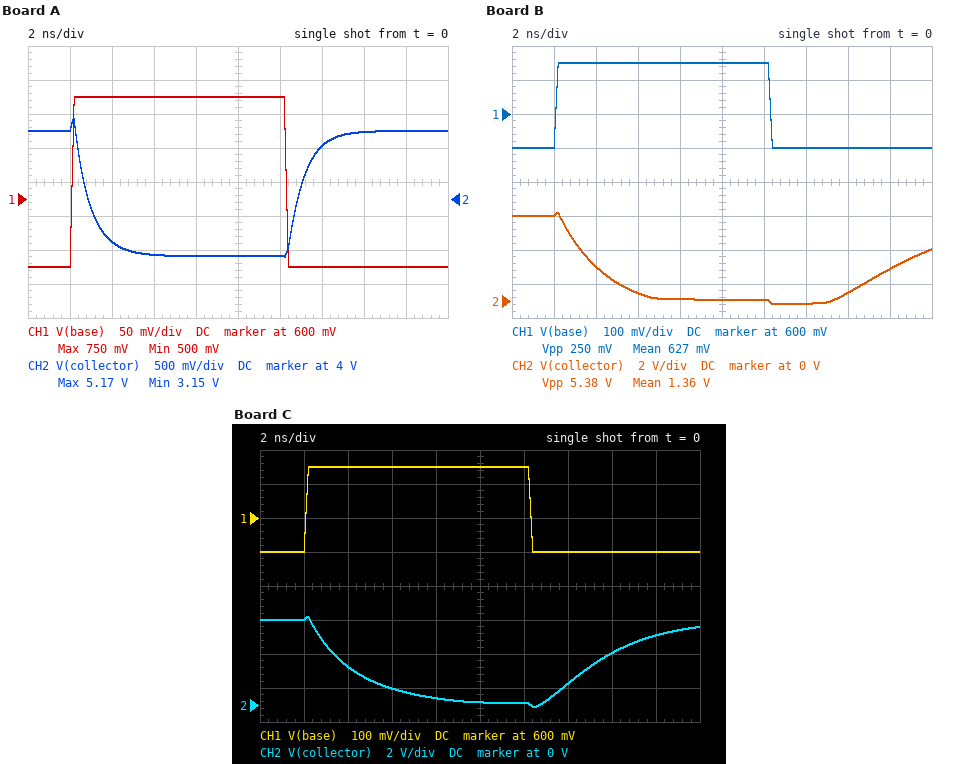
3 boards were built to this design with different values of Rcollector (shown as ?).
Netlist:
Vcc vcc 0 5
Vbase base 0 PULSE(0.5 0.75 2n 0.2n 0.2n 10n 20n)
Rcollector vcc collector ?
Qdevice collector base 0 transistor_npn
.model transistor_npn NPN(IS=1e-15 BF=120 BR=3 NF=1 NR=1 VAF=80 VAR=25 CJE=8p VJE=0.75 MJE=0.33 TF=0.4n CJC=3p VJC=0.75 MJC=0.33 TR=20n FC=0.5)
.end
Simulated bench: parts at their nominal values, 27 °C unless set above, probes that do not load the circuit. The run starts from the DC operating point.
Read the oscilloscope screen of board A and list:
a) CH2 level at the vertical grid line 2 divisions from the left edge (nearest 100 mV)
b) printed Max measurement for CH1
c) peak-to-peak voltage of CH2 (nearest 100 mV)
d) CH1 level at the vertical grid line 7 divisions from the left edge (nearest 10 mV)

3.4 V
750 mV
2.0 V
500 mV
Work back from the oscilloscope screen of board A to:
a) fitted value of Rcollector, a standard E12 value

470 Ω
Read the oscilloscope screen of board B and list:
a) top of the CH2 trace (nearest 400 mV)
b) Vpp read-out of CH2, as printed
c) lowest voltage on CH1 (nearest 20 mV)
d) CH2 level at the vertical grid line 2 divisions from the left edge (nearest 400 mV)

5.2 V
5.38 V
500 mV
2.0 V
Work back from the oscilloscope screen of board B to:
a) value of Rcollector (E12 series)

2.2 kΩ
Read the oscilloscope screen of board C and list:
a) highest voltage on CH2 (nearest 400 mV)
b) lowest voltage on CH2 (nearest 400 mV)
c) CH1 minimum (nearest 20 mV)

5.2 V
0 V
500 mV
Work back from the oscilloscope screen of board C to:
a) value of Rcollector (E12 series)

1.5 kΩ
